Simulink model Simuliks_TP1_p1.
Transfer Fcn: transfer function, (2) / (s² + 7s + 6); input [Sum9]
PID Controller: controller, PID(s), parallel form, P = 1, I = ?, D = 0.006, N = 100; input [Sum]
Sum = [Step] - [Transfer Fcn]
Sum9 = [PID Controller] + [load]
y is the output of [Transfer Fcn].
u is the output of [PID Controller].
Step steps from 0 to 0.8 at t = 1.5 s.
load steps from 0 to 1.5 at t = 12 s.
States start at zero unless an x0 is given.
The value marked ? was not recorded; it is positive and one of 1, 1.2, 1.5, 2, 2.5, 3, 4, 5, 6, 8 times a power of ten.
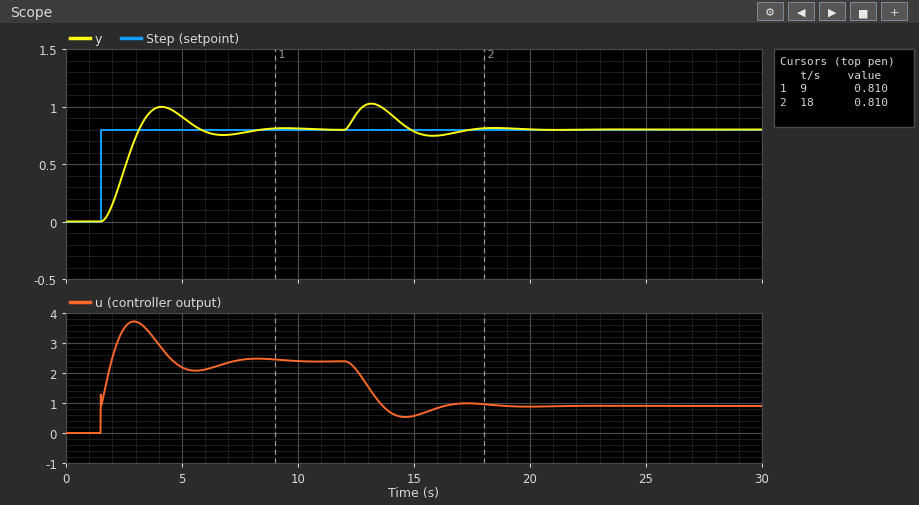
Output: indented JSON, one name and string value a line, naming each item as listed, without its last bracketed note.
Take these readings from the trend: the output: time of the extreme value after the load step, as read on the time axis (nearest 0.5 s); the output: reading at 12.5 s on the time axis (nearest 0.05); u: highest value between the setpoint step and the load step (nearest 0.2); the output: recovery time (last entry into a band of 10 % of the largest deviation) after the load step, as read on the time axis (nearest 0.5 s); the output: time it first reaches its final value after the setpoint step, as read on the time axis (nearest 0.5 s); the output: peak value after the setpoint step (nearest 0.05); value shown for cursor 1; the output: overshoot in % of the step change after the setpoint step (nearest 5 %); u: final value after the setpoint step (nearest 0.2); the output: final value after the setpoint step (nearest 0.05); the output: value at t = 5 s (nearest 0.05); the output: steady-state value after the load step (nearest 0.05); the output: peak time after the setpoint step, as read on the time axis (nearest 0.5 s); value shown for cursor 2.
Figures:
{
  "the output: time of the extreme value after the load step, as read on the time axis": "13.0 s",
  "the output: reading at 12.5 s on the time axis": "0.95",
  "u: highest value between the setpoint step and the load step": "3.8",
  "the output: recovery time (last entry into a band of 10 % of the largest deviation) after the load step, as read on the time axis": "17.0 s",
  "the output: time it first reaches its final value after the setpoint step, as read on the time axis": "3.0 s",
  "the output: peak value after the setpoint step": "1.00",
  "value shown for cursor 1": "0.810",
  "the output: overshoot in % of the step change after the setpoint step": "25 %",
  "u: final value after the setpoint step": "2.4",
  "the output: final value after the setpoint step": "0.80",
  "the output: value at t = 5 s": "0.90",
  "the output: steady-state value after the load step": "0.80",
  "the output: peak time after the setpoint step, as read on the time axis": "4.0 s",
  "value shown for cursor 2": "0.810"
}
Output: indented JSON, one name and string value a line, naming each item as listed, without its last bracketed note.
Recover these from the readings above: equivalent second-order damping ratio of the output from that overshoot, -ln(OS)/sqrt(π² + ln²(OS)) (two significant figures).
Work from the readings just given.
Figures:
{
  "equivalent second-order damping ratio of the output from that overshoot, -ln(OS)/sqrt(π² + ln²(OS))": "0.40"
}
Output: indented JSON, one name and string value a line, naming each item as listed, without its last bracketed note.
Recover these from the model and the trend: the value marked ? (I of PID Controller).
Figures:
{
  "the value marked ?": "5"
}
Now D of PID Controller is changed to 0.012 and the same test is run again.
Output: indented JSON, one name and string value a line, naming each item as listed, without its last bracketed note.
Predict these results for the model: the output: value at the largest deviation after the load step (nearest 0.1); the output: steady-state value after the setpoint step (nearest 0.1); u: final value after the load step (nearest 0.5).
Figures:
{
  "the output: value at the largest deviation after the load step": "1.0",
  "the output: steady-state value after the setpoint step": "0.8",
  "u: final value after the load step": "1.0"
}
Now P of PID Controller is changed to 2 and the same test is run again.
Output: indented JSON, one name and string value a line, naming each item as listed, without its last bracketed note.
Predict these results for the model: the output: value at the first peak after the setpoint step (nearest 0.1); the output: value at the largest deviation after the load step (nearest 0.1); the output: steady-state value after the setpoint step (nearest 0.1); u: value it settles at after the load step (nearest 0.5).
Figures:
{
  "the output: value at the first peak after the setpoint step": "0.9",
  "the output: value at the largest deviation after the load step": "1.0",
  "the output: steady-state value after the setpoint step": "0.8",
  "u: value it settles at after the load step": "1.0"
}
